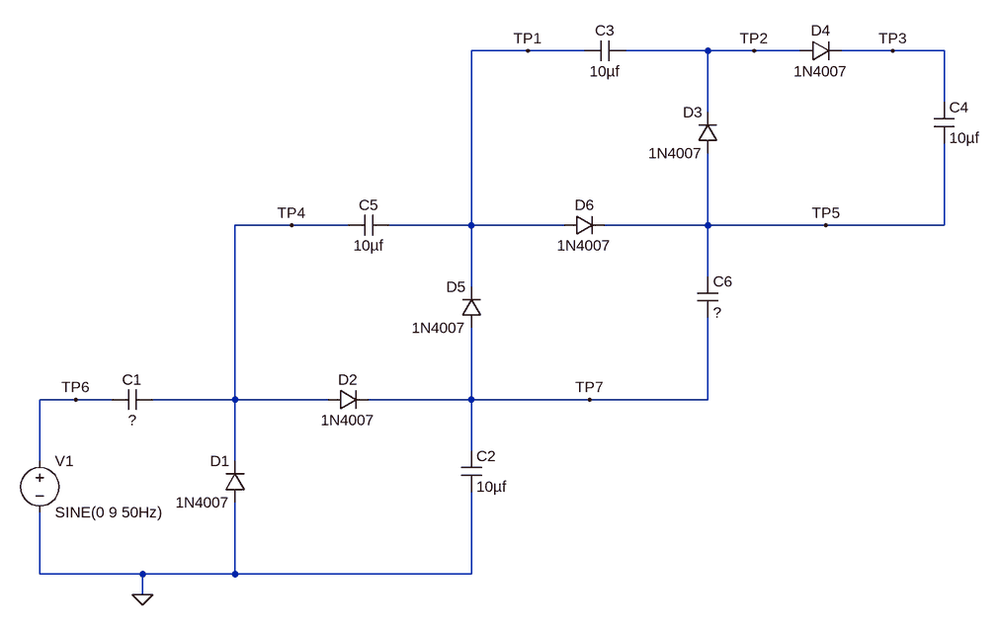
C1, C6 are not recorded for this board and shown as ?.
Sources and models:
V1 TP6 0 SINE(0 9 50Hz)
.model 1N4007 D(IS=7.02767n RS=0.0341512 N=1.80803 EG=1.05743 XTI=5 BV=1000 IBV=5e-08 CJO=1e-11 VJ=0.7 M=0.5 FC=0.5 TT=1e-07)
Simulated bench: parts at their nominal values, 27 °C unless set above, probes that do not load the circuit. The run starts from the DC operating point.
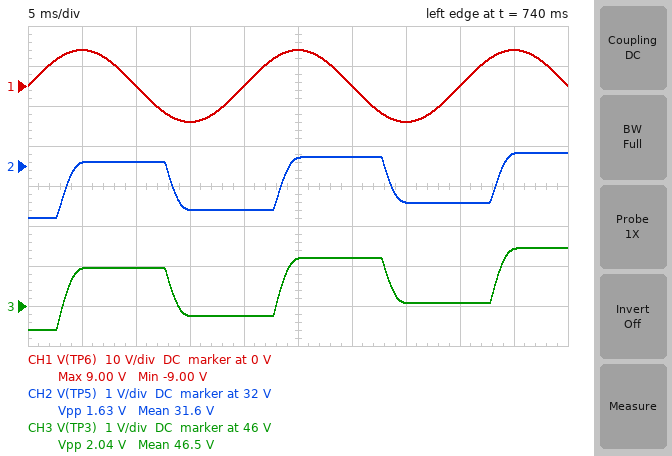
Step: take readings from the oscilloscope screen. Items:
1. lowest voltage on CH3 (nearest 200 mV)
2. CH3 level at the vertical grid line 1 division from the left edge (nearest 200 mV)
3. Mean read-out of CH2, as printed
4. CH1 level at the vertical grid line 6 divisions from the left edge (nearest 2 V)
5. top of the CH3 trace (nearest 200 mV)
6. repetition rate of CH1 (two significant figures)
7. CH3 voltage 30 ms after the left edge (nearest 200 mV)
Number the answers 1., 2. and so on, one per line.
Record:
1. 45.4 V
2. 47.0 V
3. 31.6 V
4. 0 V
5. 47.4 V
6. 50 Hz
7. 47.2 V
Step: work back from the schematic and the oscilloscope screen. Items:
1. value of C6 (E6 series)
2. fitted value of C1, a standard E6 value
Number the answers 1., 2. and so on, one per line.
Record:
1. 3.3 µF
2. 6.8 µF
